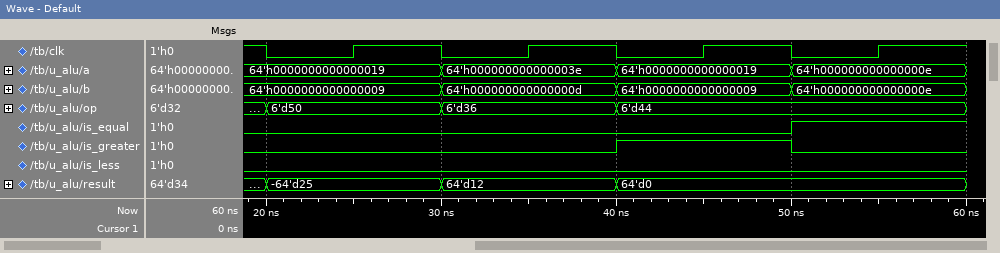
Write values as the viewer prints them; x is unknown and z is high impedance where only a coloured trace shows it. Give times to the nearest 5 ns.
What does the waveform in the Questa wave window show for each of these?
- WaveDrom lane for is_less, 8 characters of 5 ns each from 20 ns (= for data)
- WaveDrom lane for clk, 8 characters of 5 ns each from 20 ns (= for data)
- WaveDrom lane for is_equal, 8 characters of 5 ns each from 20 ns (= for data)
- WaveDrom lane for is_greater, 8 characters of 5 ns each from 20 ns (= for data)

{name: 'is_less', wave: '0.......'}
{name: 'clk', wave: '01010101'}
{name: 'is_equal', wave: '0.....1.'}
{name: 'is_greater', wave: '0...1.0.'}
